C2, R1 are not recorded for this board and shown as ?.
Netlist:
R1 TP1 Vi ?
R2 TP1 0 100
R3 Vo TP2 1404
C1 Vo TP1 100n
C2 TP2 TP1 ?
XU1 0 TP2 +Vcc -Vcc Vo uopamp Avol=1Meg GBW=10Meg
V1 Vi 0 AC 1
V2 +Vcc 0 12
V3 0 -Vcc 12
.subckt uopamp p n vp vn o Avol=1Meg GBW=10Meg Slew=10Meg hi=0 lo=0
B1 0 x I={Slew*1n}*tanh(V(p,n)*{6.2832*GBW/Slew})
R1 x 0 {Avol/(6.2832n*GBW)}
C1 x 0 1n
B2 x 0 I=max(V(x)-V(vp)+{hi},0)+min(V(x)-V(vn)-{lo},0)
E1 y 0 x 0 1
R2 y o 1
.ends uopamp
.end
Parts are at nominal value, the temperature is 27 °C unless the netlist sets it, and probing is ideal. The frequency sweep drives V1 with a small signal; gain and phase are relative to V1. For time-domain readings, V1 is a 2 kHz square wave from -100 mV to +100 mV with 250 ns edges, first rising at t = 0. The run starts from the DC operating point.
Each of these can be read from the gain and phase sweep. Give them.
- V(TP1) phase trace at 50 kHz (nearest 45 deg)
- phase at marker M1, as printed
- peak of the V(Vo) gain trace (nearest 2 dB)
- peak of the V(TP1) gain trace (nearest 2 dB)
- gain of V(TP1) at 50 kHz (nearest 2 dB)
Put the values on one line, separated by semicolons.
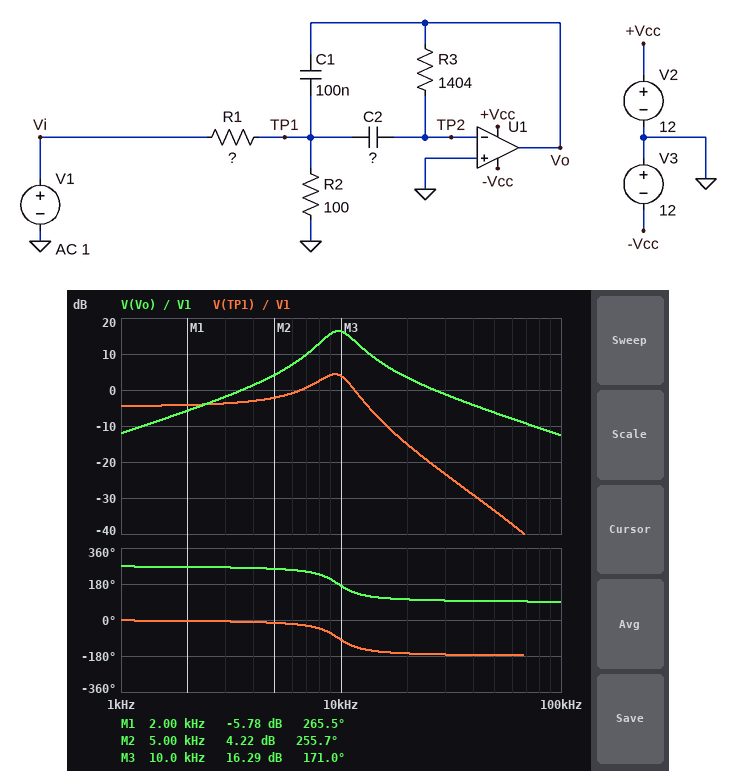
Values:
-180 deg; 265.5 deg; 16 dB; 4 dB; -34 dB
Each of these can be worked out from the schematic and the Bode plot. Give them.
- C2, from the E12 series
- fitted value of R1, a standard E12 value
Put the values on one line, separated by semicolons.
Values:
47 nF; 68 Ω
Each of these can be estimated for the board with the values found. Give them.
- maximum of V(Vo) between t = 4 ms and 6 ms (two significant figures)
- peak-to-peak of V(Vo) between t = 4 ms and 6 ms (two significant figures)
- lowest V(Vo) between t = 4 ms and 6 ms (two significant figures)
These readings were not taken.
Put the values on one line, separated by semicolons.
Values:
390 mV; 770 mV; -390 mV
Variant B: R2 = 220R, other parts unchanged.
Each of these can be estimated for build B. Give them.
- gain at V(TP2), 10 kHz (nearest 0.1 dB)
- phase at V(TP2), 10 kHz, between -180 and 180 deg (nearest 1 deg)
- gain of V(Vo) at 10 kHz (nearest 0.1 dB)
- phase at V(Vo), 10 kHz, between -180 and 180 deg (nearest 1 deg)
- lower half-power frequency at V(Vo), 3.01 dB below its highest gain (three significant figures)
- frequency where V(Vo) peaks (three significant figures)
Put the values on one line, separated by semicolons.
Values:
-45.5 dB; 54 deg; 14.5 dB; 143 deg; 7.00 kHz; 8.58 kHz
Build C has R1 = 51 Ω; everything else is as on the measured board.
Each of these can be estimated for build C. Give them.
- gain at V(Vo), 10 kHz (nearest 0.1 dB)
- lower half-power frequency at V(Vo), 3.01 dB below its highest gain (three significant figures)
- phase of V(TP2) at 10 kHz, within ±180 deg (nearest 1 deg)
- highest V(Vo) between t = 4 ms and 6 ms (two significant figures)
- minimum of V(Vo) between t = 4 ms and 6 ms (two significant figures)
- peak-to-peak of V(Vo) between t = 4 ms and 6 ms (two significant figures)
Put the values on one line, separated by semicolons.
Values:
18.3 dB; 9.02 kHz; 111 deg; 490 mV; -490 mV; 970 mV
